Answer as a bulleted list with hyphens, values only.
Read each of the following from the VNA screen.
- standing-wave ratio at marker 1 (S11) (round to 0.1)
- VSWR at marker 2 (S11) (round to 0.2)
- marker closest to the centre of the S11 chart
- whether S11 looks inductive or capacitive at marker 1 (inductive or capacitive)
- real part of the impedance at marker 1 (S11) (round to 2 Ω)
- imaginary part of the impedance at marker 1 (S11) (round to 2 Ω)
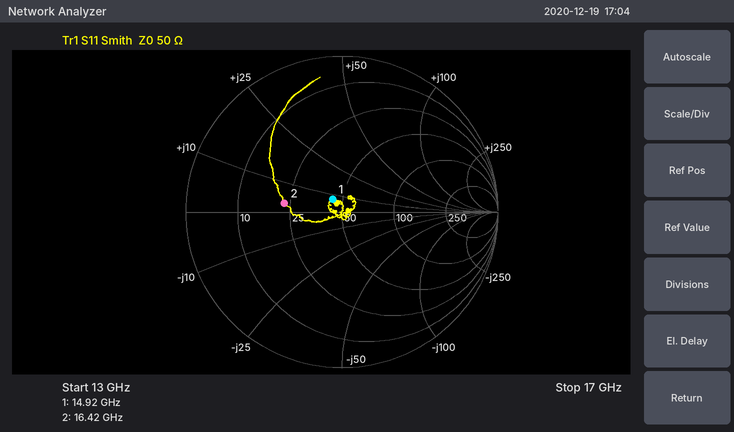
- 1.2
- 2.2
- marker 1
- inductive
- 44 Ω
- +8 Ω
